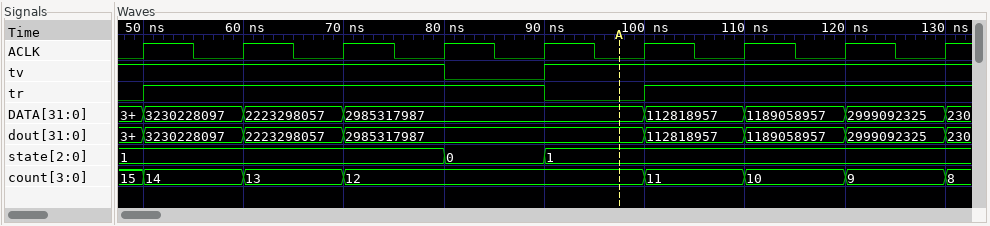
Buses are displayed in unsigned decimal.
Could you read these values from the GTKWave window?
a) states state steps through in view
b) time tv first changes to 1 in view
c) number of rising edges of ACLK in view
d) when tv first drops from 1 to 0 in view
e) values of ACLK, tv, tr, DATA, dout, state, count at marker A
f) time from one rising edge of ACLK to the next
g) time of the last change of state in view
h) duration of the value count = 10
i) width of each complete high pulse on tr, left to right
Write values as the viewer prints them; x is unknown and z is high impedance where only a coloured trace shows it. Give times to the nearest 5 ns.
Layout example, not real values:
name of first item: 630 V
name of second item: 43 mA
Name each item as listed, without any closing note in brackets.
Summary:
states state steps through in view: 1, 0, 1
time tv first changes to 1 in view: 90 ns
number of rising edges of ACLK in view: 9
when tv first drops from 1 to 0 in view: 80 ns
values of ACLK, tv, tr, DATA, dout, state, count at marker A: ACLK=0, tv=1, tr=0, DATA=2985317987, dout=2985317987, state=1, count=12
time from one rising edge of ACLK to the next: 10 ns
time of the last change of state in view: 90 ns
duration of the value count = 10: 10 ns
width of each complete high pulse on tr, left to right: 40 ns
